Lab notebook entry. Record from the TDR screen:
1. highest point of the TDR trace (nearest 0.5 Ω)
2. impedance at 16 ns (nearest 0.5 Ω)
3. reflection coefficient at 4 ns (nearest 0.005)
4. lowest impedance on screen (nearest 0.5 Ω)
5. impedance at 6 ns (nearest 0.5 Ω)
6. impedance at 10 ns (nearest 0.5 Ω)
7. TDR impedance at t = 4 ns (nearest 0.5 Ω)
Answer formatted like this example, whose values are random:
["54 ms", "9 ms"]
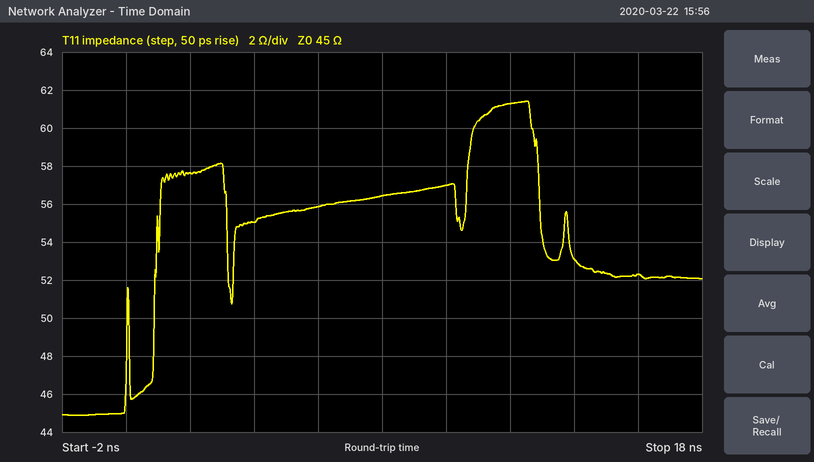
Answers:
["61.5 Ω", "52.5 Ω", "+0.100", "45.0 Ω", "56.0 Ω", "57.0 Ω", "55.0 Ω"]
